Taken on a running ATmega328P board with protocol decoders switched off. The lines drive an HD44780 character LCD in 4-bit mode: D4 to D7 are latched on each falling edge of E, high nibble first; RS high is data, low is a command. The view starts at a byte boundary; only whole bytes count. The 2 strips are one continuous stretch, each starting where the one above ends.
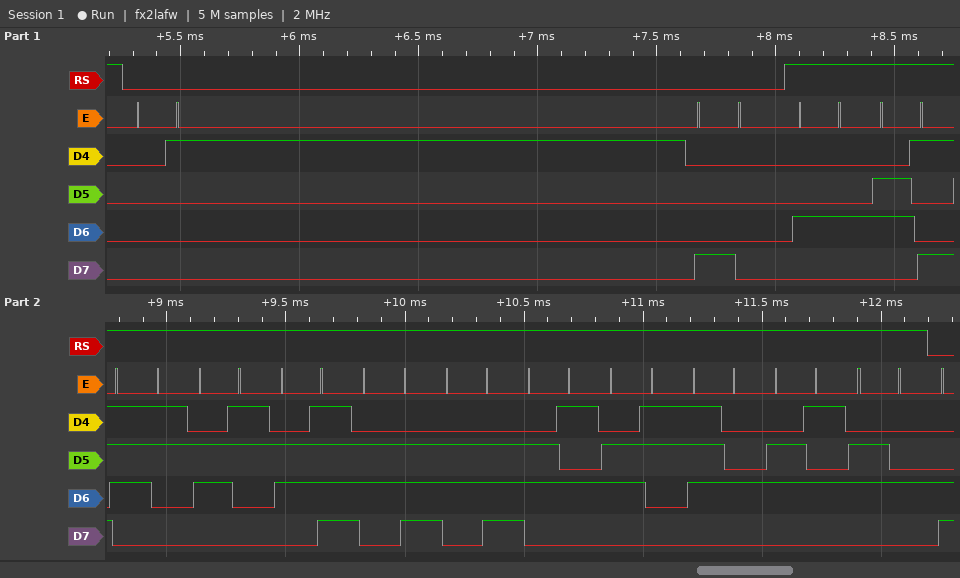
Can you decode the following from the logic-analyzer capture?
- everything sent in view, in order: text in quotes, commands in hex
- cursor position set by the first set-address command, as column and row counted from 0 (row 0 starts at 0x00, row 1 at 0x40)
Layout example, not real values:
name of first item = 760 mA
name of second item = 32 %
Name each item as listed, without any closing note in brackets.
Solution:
everything sent in view, in order: text in quotes, commands in hex = 0x01 0x80 "Disconnected"
cursor position set by the first set-address command, as column and row counted from 0 = column 0, row 0
